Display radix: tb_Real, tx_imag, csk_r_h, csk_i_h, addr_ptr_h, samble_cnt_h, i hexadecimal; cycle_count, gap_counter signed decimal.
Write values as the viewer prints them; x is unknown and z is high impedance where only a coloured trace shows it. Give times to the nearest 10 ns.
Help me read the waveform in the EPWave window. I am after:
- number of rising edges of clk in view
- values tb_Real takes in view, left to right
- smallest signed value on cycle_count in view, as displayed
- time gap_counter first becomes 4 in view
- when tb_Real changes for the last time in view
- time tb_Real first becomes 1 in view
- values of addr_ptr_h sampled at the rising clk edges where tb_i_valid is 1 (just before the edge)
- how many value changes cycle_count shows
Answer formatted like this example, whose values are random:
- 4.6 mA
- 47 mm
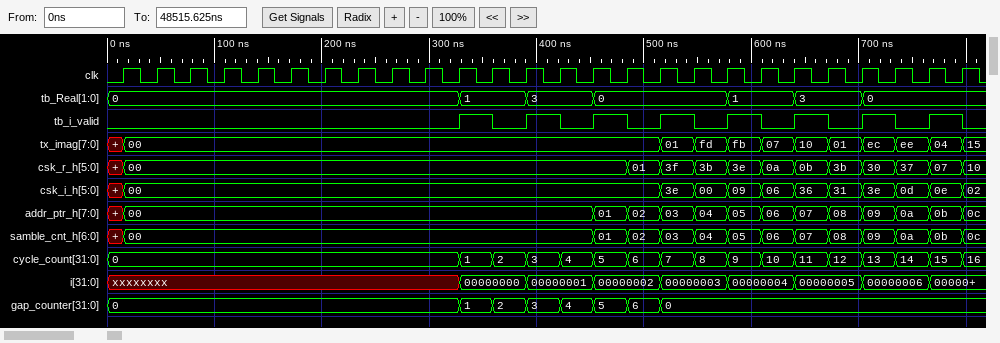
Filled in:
- 26
- 0, 1, 3, 0, 1, 3, 0
- 0
- 420 ns
- 700 ns
- 330 ns
- 00, 00, 01, 03, 05, 07, 09, 0b
- 16
